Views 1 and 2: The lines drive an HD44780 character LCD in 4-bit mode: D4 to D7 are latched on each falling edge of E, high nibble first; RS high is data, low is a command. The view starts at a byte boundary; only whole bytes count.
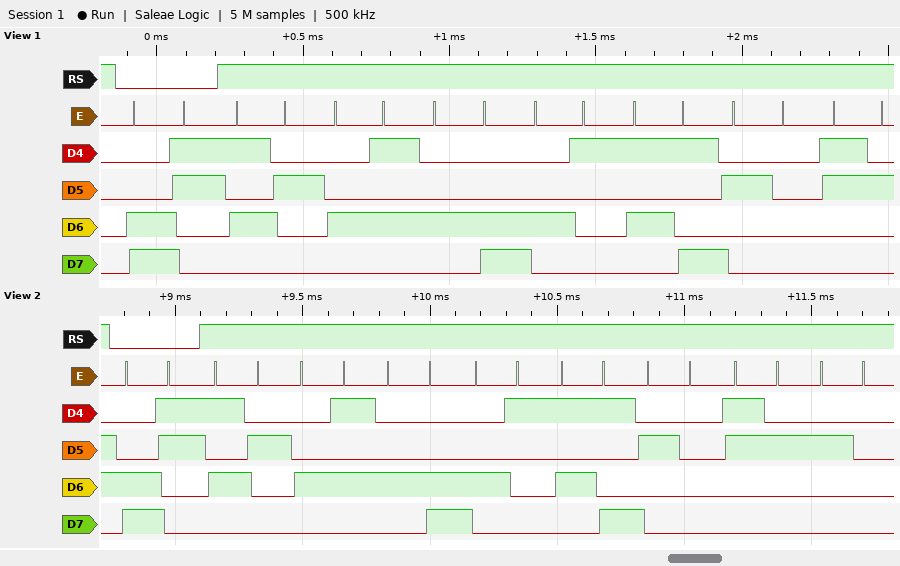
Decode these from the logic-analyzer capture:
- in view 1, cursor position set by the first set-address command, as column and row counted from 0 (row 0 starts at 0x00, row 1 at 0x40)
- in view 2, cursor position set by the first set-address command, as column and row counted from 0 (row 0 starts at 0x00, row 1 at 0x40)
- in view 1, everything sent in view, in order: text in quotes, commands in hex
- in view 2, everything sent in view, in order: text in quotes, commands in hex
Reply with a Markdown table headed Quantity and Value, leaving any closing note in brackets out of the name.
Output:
| Quantity | Value |
|---|---|
| in view 1, cursor position set by the first set-address command, as column and row counted from 0 | column 3, row 1 |
| in view 2, cursor position set by the first set-address command, as column and row counted from 0 | column 3, row 1 |
| in view 1, everything sent in view, in order: text in quotes, commands in hex | 0xC3 "RELAY 2" |
| in view 2, everything sent in view, in order: text in quotes, commands in hex | 0xC3 "RELAY 2 " |
